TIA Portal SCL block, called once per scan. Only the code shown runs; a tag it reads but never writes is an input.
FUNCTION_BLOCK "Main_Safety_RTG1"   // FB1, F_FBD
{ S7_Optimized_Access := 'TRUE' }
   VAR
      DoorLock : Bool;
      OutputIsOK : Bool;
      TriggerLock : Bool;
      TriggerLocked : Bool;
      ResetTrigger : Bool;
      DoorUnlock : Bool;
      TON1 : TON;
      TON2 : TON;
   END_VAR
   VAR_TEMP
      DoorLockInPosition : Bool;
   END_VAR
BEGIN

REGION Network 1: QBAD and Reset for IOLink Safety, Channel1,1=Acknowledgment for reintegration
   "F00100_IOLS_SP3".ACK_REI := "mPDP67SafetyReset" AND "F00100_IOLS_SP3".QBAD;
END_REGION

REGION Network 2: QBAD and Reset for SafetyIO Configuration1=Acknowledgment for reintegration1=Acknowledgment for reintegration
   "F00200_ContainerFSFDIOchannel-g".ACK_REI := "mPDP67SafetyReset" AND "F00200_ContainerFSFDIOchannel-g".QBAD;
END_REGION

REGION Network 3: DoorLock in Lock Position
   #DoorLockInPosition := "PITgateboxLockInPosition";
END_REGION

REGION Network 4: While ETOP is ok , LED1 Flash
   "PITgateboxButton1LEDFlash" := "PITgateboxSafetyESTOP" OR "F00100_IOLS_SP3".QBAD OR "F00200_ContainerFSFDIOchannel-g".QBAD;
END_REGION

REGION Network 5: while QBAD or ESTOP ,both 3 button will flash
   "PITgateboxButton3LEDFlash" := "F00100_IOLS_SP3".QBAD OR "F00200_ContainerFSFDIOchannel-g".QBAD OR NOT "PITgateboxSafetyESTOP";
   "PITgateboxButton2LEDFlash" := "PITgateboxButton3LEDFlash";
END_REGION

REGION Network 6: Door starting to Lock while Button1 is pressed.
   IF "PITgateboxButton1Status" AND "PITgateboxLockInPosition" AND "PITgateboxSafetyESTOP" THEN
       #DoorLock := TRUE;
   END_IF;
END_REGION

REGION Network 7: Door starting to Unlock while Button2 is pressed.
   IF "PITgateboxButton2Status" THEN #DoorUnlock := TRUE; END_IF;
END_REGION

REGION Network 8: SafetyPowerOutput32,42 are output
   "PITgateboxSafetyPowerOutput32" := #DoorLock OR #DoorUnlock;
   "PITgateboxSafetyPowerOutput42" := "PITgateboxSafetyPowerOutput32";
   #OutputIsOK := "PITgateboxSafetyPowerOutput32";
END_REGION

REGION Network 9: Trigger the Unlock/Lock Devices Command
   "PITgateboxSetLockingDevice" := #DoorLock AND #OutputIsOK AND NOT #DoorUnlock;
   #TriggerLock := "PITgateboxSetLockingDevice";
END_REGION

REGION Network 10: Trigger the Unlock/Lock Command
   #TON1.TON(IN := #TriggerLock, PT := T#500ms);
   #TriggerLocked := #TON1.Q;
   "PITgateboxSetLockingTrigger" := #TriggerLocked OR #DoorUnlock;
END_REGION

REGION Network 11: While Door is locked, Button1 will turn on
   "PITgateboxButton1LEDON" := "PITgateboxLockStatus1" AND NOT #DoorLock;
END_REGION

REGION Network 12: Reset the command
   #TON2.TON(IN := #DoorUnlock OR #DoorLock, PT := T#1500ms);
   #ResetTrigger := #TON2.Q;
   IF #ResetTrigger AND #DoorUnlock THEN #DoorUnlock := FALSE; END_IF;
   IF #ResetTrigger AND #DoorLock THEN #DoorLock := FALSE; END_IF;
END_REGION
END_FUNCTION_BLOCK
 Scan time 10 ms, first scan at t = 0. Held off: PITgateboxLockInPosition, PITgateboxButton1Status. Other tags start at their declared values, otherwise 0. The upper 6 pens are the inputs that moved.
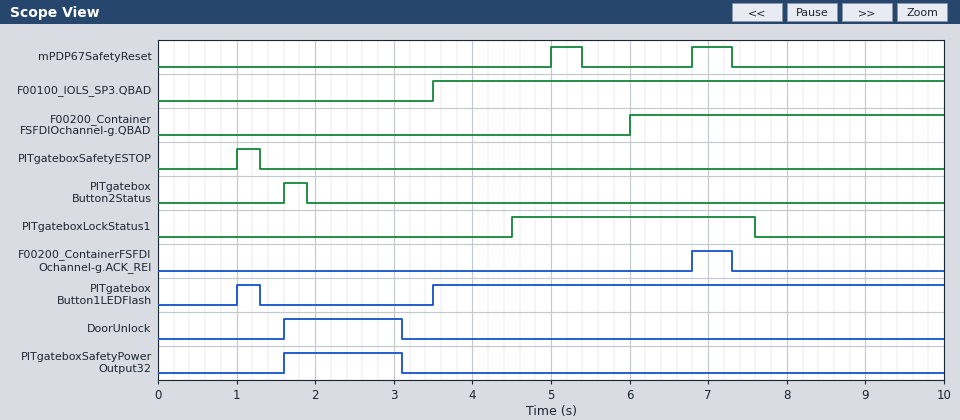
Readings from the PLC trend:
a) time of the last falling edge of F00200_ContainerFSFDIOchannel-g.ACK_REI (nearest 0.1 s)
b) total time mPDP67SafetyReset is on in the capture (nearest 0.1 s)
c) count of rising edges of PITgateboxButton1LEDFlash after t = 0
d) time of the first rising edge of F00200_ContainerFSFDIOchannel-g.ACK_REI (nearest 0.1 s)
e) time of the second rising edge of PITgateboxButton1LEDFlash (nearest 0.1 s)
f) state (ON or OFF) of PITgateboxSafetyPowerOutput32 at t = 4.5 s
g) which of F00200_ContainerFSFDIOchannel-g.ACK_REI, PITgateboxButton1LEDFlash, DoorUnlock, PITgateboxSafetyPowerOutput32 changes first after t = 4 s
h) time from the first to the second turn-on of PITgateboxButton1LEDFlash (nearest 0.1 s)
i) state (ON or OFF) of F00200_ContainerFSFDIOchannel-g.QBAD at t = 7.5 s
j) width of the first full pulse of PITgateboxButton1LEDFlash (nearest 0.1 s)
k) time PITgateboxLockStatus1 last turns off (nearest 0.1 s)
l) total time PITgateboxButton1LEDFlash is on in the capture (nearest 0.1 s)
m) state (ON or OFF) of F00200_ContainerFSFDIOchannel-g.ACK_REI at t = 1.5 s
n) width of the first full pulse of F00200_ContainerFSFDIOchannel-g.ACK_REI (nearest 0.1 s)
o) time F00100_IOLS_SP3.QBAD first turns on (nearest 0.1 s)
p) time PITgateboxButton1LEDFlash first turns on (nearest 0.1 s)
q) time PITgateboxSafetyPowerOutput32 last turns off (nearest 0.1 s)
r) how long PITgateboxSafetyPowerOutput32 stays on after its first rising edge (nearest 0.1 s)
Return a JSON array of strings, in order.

["7.3 s", "0.9 s", "2", "6.8 s", "3.5 s", "OFF", "F00200_ContainerFSFDIOchannel-g.ACK_REI", "2.5 s", "ON", "0.3 s", "7.6 s", "6.8 s", "OFF", "0.5 s", "3.5 s", "1.0 s", "3.1 s", "1.5 s"]
